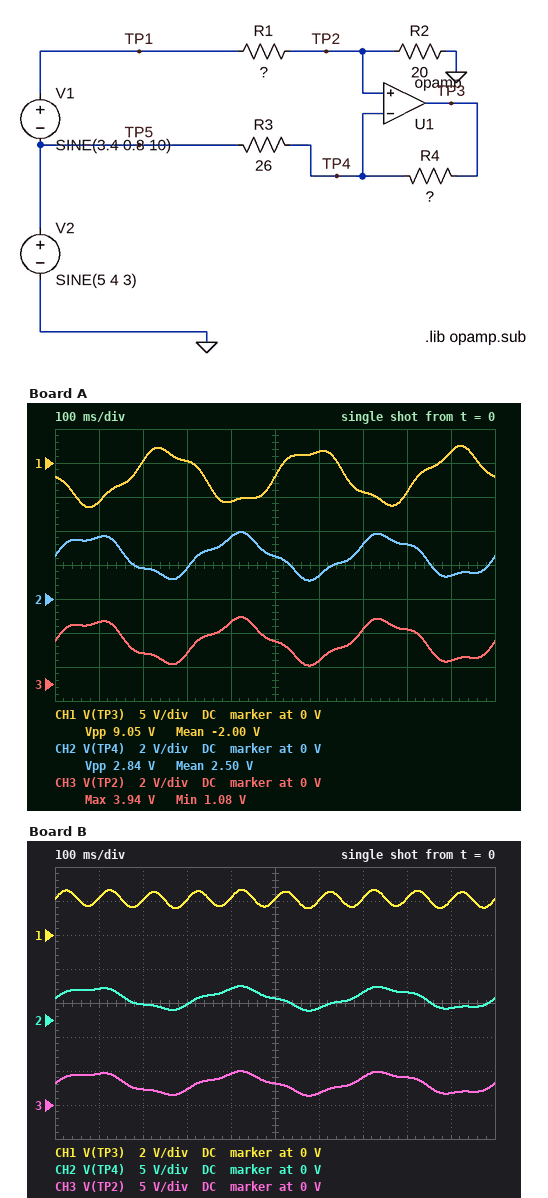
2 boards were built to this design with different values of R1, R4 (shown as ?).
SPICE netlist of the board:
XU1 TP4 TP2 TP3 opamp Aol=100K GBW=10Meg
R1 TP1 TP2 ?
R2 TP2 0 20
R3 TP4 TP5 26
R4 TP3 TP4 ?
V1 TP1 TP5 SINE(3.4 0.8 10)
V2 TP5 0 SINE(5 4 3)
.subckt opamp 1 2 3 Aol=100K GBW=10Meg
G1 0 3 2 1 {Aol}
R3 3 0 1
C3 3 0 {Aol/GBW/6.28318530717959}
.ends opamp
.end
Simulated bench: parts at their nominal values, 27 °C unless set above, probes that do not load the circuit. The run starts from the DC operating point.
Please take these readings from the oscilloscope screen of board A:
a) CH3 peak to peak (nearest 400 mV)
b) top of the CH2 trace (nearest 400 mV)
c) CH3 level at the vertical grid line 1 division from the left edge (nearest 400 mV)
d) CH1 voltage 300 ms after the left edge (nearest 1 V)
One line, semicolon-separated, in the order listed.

2.8 V; 4.0 V; 3.6 V; 0 V
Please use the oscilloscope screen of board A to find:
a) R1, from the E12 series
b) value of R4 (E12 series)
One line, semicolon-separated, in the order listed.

47 Ω; 47 Ω
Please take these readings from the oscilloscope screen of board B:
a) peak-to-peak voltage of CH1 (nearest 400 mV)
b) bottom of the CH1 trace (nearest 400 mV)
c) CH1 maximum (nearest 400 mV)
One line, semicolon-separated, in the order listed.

1.2 V; 1.6 V; 2.8 V
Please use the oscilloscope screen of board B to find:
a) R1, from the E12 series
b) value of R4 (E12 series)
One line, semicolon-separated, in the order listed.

33 Ω; 15 Ω
